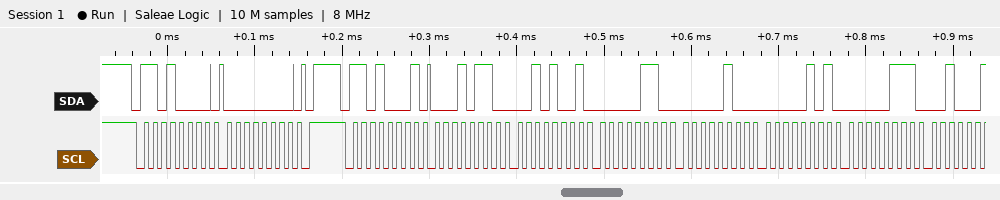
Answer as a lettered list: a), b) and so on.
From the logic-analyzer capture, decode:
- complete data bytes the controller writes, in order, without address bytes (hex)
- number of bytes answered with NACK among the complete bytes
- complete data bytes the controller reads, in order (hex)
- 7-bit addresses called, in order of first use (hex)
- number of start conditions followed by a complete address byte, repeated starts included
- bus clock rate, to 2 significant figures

a) 00
b) 0
c) 16 29 06 04 05 07
d) 0x68
e) 2
f) 100 kHz
